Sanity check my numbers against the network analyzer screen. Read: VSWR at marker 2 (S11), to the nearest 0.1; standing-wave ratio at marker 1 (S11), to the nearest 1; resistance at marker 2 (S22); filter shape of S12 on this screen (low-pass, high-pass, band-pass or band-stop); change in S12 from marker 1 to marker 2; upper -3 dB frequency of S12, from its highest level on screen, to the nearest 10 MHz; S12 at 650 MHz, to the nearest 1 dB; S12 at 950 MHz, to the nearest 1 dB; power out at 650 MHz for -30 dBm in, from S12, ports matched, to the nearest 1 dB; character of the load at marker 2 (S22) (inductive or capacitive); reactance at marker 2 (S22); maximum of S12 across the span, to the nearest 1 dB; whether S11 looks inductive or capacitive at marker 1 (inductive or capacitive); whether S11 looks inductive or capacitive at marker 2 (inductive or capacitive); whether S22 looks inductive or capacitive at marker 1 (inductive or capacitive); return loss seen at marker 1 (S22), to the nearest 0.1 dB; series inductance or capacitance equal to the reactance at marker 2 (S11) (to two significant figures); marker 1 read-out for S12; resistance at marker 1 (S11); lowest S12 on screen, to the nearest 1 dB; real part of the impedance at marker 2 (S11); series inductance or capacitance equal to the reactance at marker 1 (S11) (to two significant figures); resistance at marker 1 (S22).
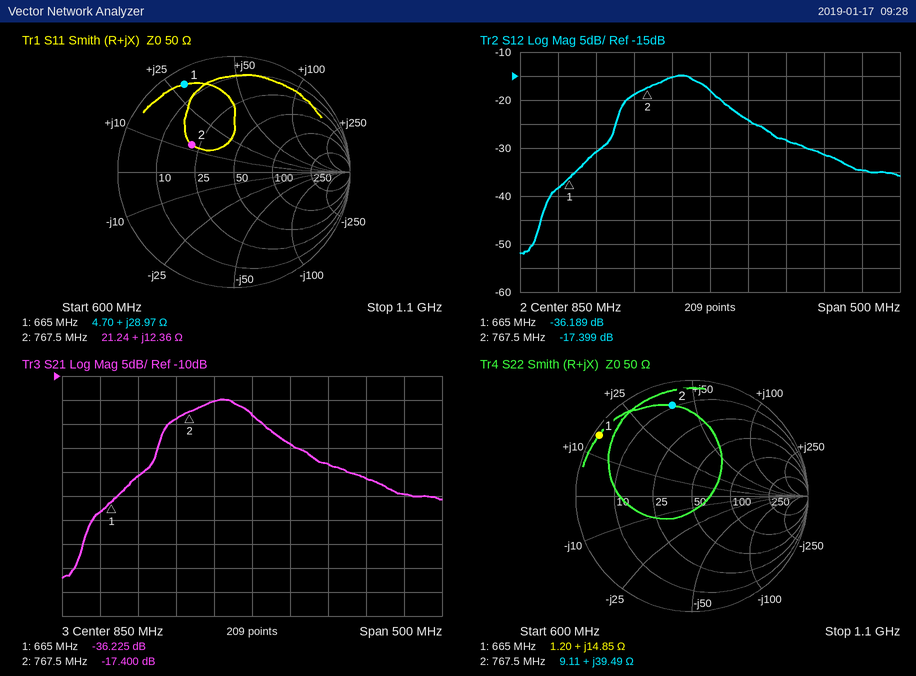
2.5
14
9.11 Ω
band-pass
18.790 dB
850 MHz
-38 dB
-28 dB
-68 dBm
inductive
+39.49 Ω
-15 dB
inductive
inductive
inductive
0.4 dB
2.6 nH
-36.189 dB
4.70 Ω
-52 dB
21.24 Ω
6.9 nH
1.20 Ω
